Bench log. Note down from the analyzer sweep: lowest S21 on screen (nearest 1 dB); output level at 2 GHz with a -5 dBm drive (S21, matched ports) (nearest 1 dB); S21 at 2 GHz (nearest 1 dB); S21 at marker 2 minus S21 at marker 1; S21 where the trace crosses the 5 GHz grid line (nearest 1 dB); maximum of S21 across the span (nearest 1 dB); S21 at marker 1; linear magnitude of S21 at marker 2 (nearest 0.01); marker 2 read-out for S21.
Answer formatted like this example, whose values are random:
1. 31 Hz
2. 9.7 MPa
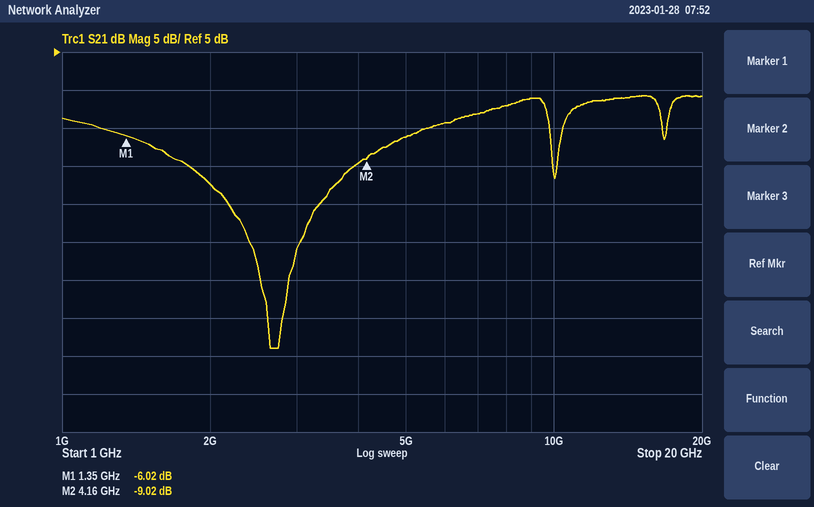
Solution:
1. -34 dB
2. -17 dBm
3. -12 dB
4. -3.00 dB
5. -6 dB
6. -1 dB
7. -6.02 dB
8. 0.35
9. -9.02 dB
